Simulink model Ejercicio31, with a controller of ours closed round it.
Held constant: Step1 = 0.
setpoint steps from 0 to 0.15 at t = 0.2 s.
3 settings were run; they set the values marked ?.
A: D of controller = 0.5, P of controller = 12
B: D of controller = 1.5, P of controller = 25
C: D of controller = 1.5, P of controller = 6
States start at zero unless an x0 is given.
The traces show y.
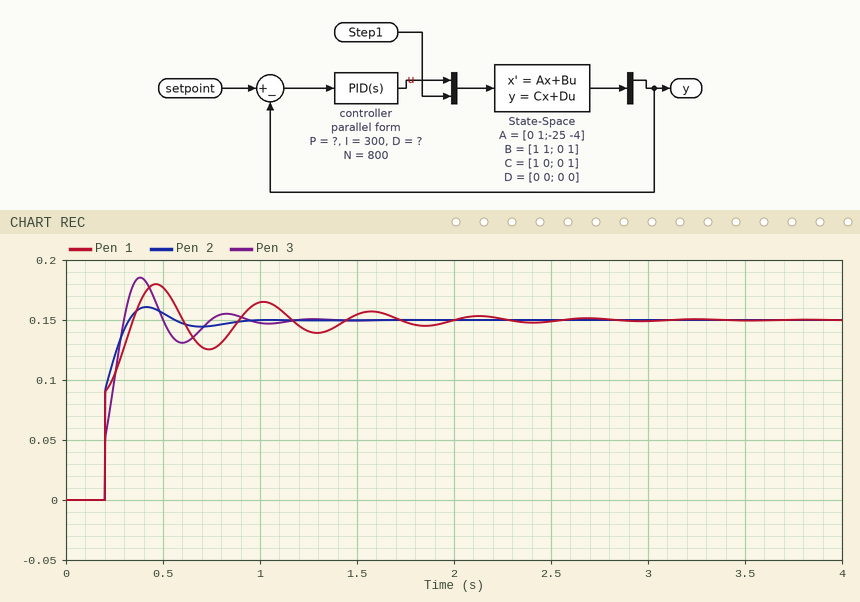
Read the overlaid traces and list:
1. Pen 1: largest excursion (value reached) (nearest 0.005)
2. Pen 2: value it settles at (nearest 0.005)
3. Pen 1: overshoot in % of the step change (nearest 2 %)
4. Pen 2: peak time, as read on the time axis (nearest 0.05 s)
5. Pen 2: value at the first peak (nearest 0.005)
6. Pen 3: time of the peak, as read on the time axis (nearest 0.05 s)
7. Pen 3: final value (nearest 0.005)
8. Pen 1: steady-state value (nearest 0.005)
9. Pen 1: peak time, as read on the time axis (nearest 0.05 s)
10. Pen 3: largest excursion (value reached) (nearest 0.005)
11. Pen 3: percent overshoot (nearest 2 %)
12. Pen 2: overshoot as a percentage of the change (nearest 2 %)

0.180
0.150
20 %
0.40 s
0.160
0.40 s
0.150
0.150
0.45 s
0.185
24 %
8 %
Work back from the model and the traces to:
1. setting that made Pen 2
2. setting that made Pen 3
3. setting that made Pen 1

B
A
C
